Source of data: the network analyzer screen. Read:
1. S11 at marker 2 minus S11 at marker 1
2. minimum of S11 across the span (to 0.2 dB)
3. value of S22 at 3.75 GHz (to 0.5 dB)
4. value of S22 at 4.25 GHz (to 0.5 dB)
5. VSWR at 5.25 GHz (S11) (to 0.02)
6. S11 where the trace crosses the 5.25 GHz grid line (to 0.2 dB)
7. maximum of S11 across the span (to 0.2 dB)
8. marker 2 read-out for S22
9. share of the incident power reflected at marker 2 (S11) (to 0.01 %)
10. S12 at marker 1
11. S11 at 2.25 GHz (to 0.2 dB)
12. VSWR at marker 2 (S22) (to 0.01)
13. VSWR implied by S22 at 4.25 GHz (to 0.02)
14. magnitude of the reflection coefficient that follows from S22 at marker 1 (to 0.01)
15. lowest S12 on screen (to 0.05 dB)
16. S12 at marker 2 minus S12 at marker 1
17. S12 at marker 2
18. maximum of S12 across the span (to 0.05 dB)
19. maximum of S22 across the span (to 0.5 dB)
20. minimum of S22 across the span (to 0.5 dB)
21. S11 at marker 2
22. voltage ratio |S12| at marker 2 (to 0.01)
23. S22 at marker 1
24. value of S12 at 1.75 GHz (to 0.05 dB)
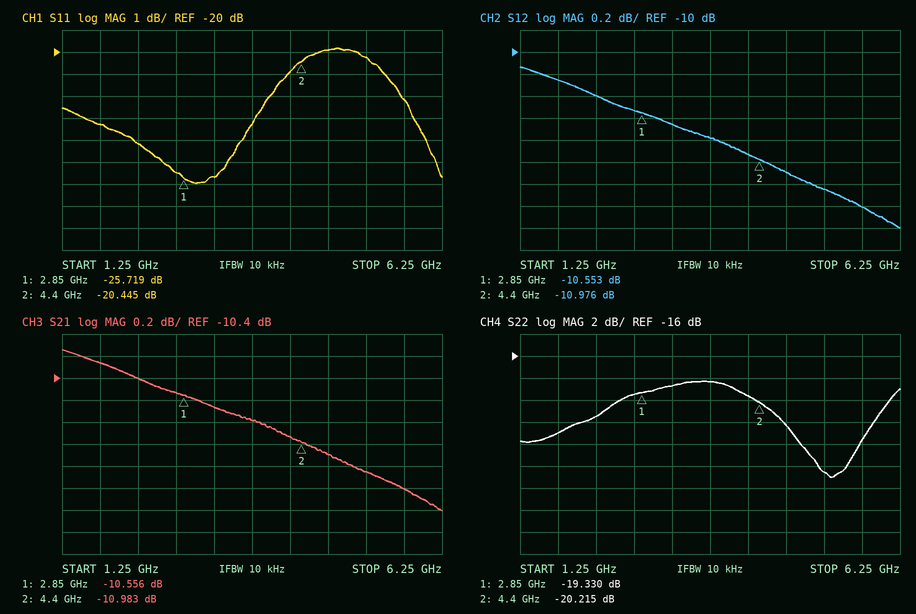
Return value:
5.274 dB
-26.0 dB
-18.5 dB
-19.5 dB
1.22
-20.2 dB
-19.8 dB
-20.215 dB
0.90 %
-10.553 dB
-24.2 dB
1.22
1.24
0.11
-11.60 dB
-0.423 dB
-10.976 dB
-10.15 dB
-18.5 dB
-27.0 dB
-20.445 dB
0.28
-19.330 dB
-10.25 dB
